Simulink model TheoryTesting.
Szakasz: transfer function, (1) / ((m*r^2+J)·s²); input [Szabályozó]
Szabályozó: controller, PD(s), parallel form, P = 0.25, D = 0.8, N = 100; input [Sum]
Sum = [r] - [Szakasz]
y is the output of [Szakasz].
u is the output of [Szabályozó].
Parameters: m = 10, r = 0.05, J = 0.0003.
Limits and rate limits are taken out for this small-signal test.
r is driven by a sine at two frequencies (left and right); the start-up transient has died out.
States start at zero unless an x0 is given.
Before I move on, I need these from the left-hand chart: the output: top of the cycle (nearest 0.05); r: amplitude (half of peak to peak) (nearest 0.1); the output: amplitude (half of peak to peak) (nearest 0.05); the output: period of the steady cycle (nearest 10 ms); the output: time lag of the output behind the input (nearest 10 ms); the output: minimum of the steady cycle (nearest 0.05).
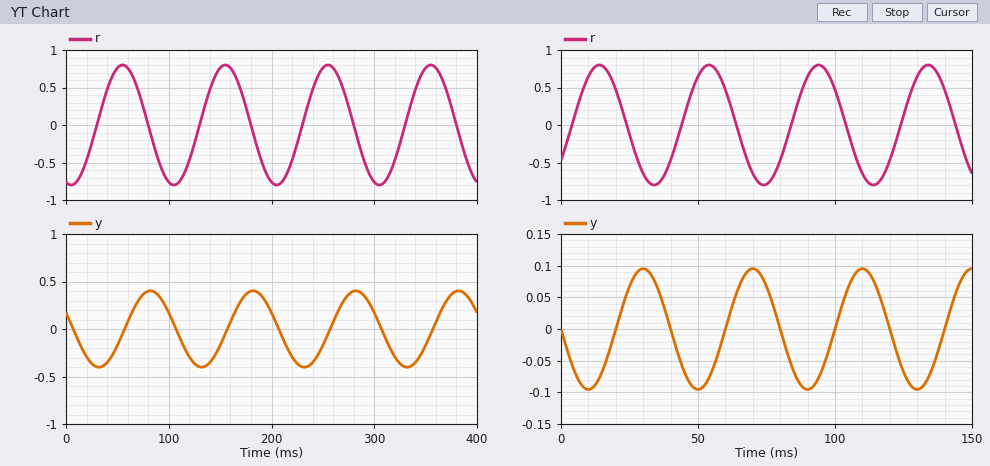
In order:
0.40
0.8
0.40
100 ms
30 ms
-0.40
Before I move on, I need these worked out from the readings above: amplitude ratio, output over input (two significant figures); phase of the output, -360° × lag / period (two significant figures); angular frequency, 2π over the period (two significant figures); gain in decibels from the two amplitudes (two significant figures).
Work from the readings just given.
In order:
0.50
-110°
0.063 rad/ms
-6.0 dB
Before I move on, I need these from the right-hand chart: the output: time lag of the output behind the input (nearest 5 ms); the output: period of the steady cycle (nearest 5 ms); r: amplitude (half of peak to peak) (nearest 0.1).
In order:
15 ms
40 ms
0.8
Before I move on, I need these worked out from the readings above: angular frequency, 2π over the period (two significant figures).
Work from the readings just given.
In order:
0.16 rad/ms
